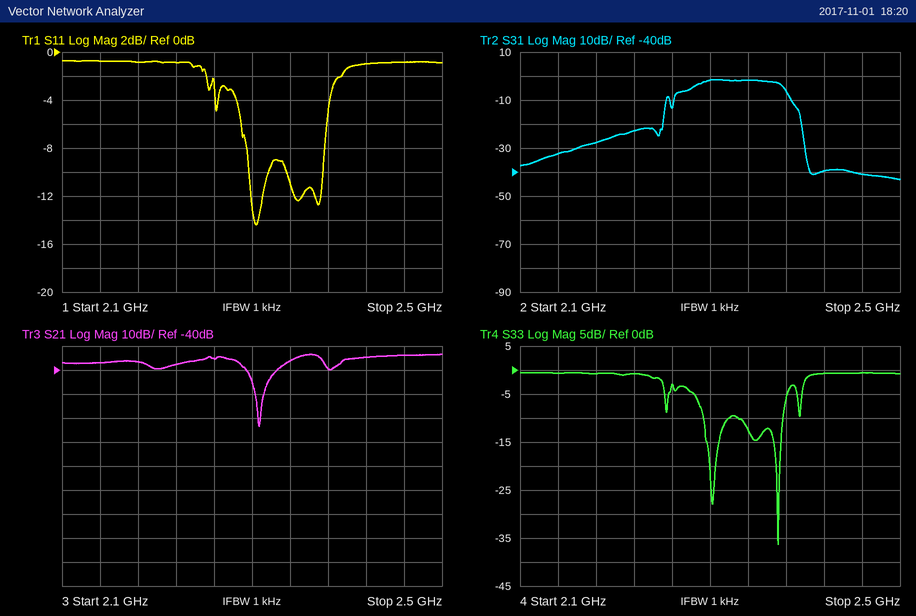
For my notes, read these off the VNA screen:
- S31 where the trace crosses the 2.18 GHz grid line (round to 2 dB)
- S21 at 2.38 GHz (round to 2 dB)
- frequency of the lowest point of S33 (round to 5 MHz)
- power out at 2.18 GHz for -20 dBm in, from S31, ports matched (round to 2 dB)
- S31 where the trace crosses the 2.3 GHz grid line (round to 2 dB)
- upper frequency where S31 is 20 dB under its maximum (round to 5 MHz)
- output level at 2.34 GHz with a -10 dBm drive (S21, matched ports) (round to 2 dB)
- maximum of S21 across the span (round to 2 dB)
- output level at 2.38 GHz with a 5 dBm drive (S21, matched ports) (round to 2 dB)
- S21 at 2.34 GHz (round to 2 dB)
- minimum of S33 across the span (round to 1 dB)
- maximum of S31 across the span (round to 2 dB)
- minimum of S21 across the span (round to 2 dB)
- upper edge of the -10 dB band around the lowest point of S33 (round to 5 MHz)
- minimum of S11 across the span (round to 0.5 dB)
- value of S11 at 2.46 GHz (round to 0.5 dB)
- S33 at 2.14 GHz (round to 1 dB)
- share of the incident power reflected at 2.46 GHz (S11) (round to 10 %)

-28 dB
-40 dB
2.370 GHz
-48 dBm
-2 dB
2.395 GHz
-46 dBm
-34 dB
-34 dBm
-36 dB
-36 dB
-2 dB
-64 dB
2.375 GHz
-14.5 dB
-1.0 dB
-1 dB
80 %
